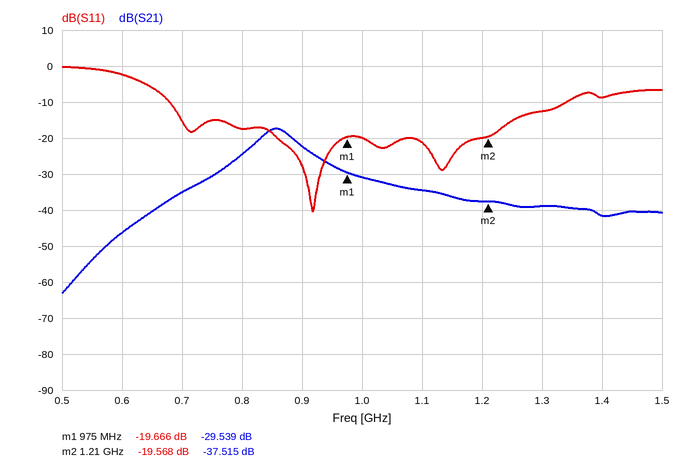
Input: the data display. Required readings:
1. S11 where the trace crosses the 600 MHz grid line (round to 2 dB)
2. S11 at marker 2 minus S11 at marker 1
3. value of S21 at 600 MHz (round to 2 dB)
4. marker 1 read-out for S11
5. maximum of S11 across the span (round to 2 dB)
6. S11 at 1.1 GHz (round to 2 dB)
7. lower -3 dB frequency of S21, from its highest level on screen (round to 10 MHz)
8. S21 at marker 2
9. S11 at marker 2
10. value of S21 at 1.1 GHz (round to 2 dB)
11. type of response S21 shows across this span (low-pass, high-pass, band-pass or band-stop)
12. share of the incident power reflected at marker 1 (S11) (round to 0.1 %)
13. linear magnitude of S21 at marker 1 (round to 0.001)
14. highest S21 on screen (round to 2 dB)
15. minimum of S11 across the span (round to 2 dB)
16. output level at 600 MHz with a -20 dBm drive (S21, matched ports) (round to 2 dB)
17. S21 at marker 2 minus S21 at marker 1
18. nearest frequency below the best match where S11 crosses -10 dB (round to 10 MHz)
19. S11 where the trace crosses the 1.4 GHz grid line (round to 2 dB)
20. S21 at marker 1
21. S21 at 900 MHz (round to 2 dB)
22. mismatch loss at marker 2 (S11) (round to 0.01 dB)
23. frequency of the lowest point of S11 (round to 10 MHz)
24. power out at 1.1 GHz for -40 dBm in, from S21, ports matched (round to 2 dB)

-2 dB
0.098 dB
-46 dB
-19.666 dB
0 dB
-22 dB
830 MHz
-37.515 dB
-19.568 dB
-34 dB
band-pass
1.1 %
0.033
-18 dB
-40 dB
-66 dBm
-7.976 dB
680 MHz
-8 dB
-29.539 dB
-22 dB
0.05 dB
920 MHz
-74 dBm
